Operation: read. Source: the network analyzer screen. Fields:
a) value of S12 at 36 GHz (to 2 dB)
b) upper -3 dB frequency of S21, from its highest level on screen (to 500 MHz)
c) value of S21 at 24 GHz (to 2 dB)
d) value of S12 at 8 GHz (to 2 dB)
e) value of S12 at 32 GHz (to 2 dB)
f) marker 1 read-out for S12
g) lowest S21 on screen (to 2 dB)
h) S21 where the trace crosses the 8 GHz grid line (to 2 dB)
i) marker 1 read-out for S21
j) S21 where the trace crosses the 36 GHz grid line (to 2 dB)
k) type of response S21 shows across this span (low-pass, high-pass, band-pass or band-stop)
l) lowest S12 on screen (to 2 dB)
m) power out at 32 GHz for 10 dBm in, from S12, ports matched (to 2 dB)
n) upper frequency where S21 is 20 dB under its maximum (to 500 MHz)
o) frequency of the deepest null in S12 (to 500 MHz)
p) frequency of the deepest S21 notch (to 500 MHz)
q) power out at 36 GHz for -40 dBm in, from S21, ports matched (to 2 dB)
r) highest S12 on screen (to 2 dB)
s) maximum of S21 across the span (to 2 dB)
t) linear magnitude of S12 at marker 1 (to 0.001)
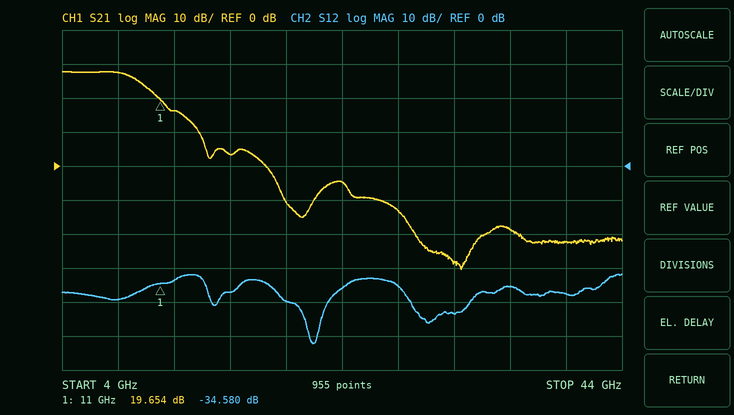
-36 dB
9.5 GHz
-4 dB
-40 dB
-44 dB
-34.580 dB
-30 dB
28 dB
19.654 dB
-18 dB
low-pass
-52 dB
-34 dBm
14.0 GHz
22.0 GHz
32.5 GHz
-58 dBm
-32 dB
28 dB
0.019
